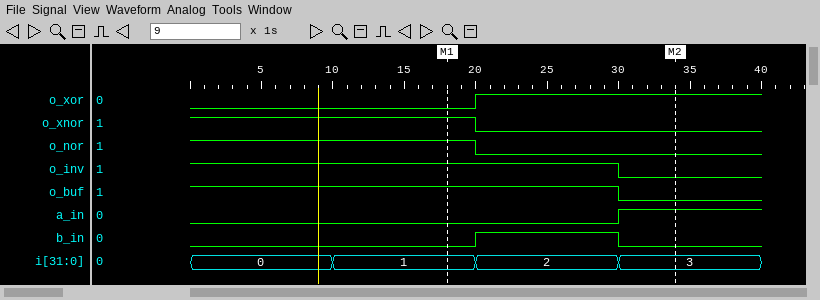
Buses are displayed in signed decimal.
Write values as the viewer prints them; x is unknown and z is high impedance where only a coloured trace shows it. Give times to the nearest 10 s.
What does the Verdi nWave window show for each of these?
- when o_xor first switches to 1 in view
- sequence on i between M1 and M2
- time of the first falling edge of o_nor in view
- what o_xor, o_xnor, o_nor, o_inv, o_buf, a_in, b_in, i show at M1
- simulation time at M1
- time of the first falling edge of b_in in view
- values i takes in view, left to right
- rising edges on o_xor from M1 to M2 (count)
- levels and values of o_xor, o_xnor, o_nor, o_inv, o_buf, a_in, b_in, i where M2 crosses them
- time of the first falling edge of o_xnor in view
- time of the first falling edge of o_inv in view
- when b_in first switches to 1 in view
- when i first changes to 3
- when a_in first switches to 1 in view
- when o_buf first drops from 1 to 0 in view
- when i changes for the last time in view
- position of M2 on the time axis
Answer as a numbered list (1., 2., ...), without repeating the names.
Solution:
1. 20 s
2. 1, 2, 3
3. 20 s
4. o_xor=0, o_xnor=1, o_nor=1, o_inv=1, o_buf=1, a_in=0, b_in=0, i=1
5. 20 s
6. 30 s
7. 0, 1, 2, 3
8. 1
9. o_xor=1, o_xnor=0, o_nor=0, o_inv=0, o_buf=0, a_in=1, b_in=0, i=3
10. 20 s
11. 30 s
12. 20 s
13. 30 s
14. 30 s
15. 30 s
16. 30 s
17. 30 s
